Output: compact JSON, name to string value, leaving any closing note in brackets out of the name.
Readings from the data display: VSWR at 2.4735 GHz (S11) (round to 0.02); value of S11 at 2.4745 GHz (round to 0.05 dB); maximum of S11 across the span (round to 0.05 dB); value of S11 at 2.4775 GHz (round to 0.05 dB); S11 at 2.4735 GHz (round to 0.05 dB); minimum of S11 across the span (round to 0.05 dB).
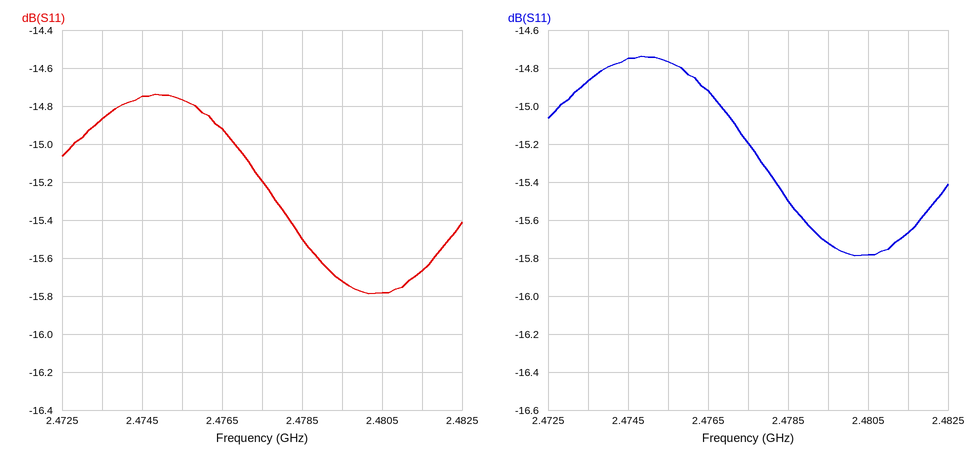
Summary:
{"VSWR at 2.4735 GHz (S11)": "1.44", "value of S11 at 2.4745 GHz": "-14.75 dB", "maximum of S11 across the span": "-14.75 dB", "value of S11 at 2.4775 GHz": "-15.20 dB", "S11 at 2.4735 GHz": "-14.85 dB", "minimum of S11 across the span": "-15.80 dB"}
